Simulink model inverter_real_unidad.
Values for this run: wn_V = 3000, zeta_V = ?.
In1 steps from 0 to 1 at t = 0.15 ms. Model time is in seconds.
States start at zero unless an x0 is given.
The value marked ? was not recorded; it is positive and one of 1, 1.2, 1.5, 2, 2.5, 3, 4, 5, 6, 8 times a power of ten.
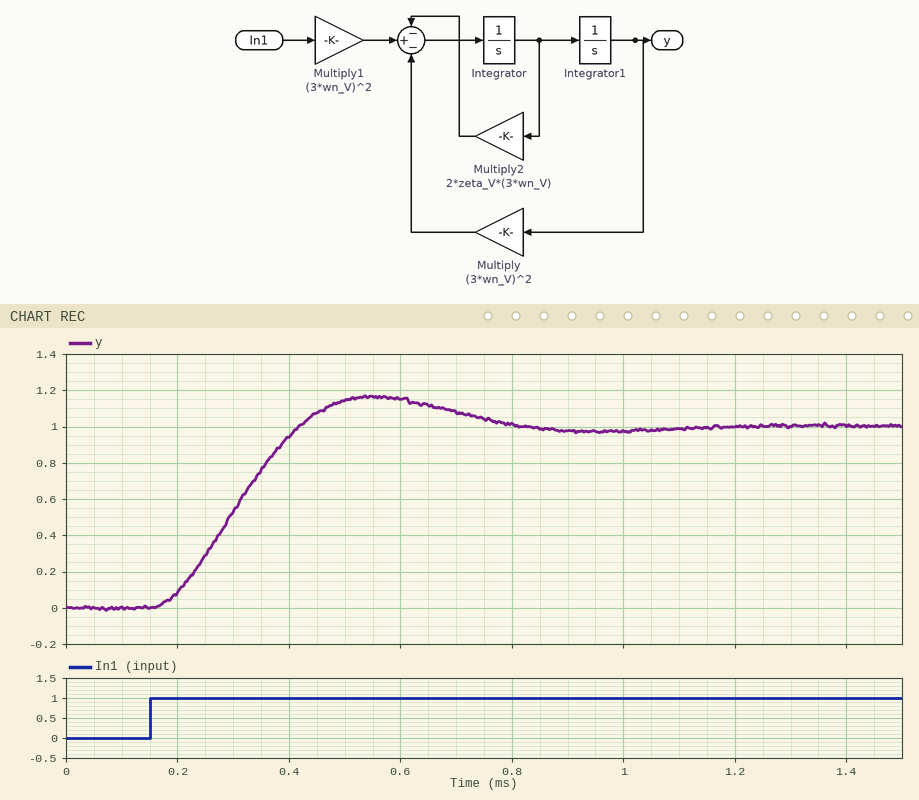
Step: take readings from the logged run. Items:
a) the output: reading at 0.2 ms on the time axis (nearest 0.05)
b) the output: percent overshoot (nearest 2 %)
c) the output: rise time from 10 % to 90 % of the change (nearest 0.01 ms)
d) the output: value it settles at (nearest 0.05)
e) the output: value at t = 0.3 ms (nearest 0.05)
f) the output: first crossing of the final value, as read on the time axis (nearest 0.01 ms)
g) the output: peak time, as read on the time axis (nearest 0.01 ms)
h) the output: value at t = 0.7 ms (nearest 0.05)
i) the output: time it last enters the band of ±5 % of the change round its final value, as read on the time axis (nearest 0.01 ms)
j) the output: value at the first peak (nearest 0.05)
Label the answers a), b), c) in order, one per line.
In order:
a) 0.10
b) 16 %
c) 0.18 ms
d) 1.00
e) 0.55
f) 0.42 ms
g) 0.55 ms
h) 1.10
i) 0.74 ms
j) 1.15
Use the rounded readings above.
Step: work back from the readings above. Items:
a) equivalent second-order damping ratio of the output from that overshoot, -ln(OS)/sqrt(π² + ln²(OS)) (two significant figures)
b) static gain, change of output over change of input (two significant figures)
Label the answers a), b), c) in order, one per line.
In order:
a) 0.50
b) 1.0
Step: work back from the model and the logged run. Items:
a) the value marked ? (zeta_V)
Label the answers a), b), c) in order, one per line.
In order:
a) 0.5
